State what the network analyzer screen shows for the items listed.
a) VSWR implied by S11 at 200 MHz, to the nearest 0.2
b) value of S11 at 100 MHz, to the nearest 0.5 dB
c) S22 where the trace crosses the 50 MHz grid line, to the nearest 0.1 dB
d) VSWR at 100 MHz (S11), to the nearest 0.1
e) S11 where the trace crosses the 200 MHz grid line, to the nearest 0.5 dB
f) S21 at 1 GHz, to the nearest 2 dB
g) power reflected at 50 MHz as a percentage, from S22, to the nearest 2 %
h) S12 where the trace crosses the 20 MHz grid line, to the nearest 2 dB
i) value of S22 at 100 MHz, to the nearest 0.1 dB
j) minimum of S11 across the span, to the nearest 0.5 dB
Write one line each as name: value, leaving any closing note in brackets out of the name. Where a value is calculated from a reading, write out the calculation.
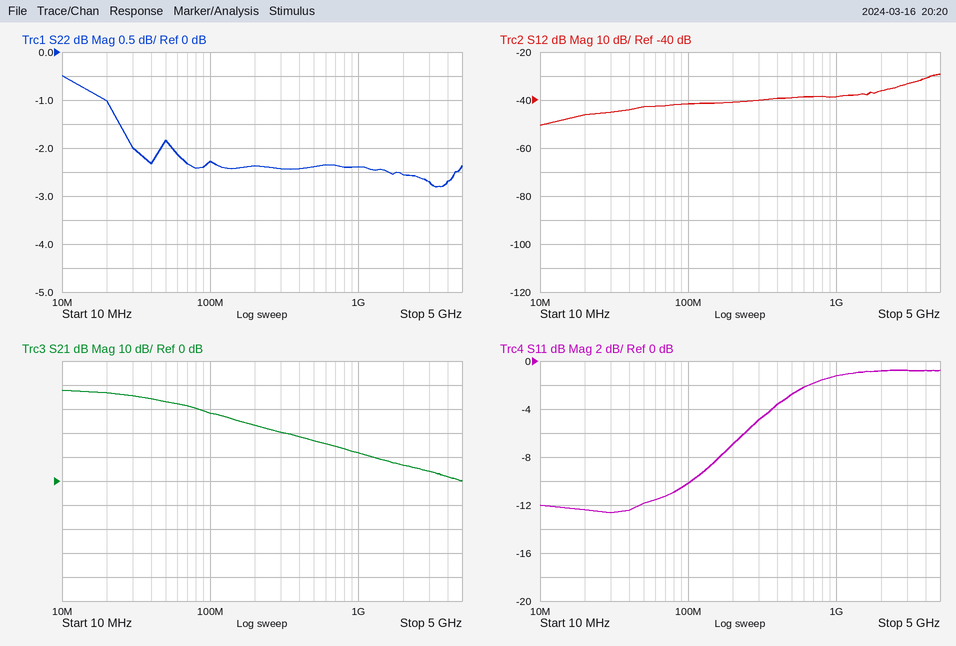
VSWR implied by S11 at 200 MHz, to the nearest 0.2: |Γ| = 10^(-7/20) = 0.4467; VSWR = (1 + 0.4467)/(1 − 0.4467) ≈ 2.6
value of S11 at 100 MHz, to the nearest 0.5 dB: -10.0 dB
S22 where the trace crosses the 50 MHz grid line, to the nearest 0.1 dB: -1.8 dB
VSWR at 100 MHz (S11), to the nearest 0.1: |Γ| = 10^(-10/20) = 0.3162; VSWR = (1 + 0.3162)/(1 − 0.3162) ≈ 1.9
S11 where the trace crosses the 200 MHz grid line, to the nearest 0.5 dB: -7.0 dB
S21 at 1 GHz, to the nearest 2 dB: 12 dB
power reflected at 50 MHz as a percentage, from S22, to the nearest 2 %: 10^(-1.8/10) ≈ 66 %
S12 where the trace crosses the 20 MHz grid line, to the nearest 2 dB: -46 dB
value of S22 at 100 MHz, to the nearest 0.1 dB: -2.3 dB
minimum of S11 across the span, to the nearest 0.5 dB: -12.5 dB
